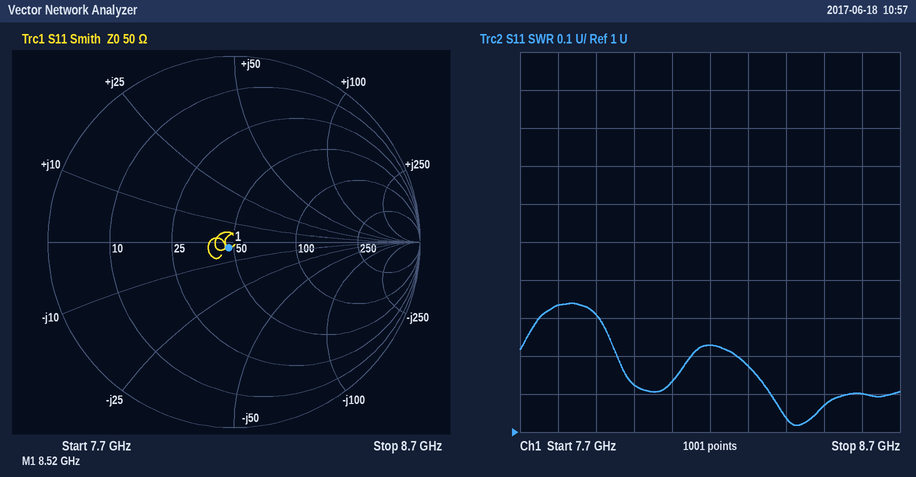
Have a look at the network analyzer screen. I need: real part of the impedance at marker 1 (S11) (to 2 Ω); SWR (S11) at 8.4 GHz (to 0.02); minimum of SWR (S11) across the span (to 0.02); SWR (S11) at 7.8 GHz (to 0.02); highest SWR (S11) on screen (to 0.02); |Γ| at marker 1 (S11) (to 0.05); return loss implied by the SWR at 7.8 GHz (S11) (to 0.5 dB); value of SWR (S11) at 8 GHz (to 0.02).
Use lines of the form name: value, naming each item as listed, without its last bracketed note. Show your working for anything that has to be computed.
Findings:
real part of the impedance at marker 1 (S11): 48 Ω
SWR (S11) at 8.4 GHz: 1.04
minimum of SWR (S11) across the span: 1.02
SWR (S11) at 7.8 GHz: 1.34
highest SWR (S11) on screen: 1.34
|Γ| at marker 1 (S11): 0.05
return loss implied by the SWR at 7.8 GHz (S11): −20 log10((1.34 − 1)/(1.34 + 1)) ≈ 16.8 dB, so 17.0 dB to the nearest 0.5 dB
value of SWR (S11) at 8 GHz: 1.12
